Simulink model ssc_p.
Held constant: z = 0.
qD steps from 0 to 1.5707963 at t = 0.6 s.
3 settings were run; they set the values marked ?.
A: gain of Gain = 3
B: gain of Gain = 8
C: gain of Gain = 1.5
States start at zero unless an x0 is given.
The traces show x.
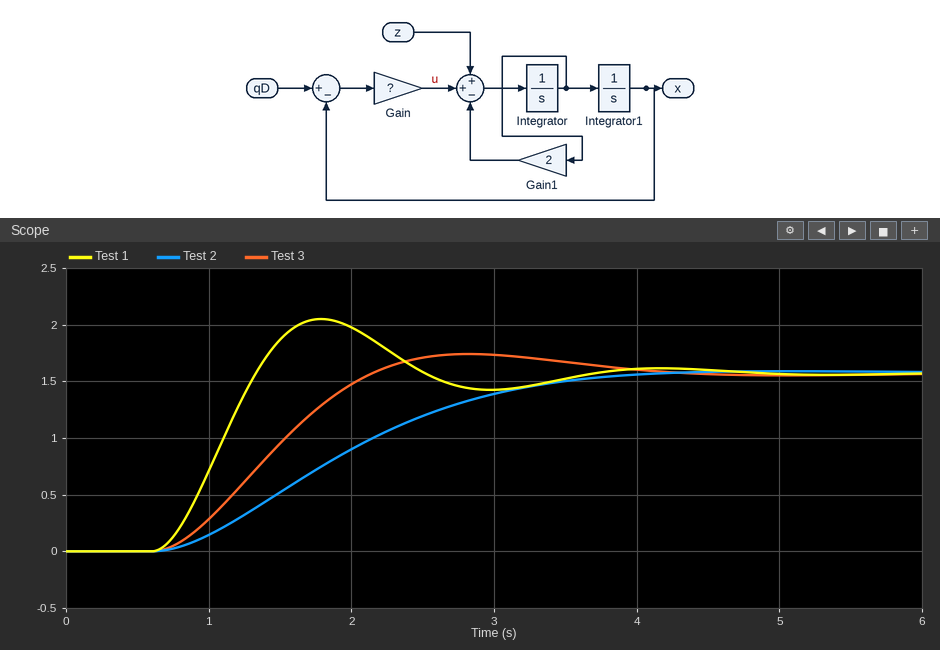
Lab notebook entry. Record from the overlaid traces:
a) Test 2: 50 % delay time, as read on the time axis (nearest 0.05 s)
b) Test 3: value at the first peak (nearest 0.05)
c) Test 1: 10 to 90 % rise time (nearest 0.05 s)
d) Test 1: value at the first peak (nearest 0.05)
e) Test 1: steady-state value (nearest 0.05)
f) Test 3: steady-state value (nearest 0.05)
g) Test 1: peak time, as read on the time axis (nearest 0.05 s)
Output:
1.85 s
1.75
0.50 s
2.05
1.55
1.55
1.80 s
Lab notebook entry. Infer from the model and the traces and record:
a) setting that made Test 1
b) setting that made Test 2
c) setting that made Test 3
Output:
B
C
A
